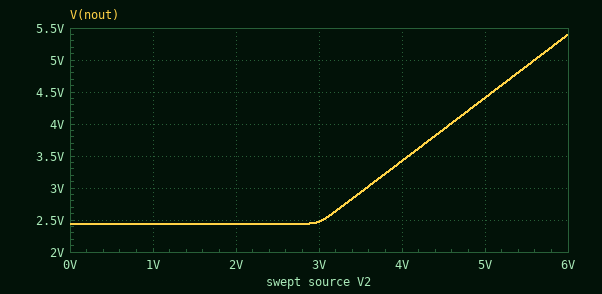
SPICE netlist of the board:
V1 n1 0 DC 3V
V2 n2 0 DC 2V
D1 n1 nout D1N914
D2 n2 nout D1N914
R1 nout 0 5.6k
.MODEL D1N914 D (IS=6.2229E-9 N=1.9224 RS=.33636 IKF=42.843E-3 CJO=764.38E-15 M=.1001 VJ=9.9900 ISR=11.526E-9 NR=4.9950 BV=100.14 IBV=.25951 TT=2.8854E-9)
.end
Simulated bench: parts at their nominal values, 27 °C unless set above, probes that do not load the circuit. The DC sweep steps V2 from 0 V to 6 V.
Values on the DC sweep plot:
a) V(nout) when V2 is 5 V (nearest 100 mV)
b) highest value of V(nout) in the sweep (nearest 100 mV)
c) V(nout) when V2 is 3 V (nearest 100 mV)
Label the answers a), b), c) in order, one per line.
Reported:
a) 4.4 V
b) 5.4 V
c) 2.5 V
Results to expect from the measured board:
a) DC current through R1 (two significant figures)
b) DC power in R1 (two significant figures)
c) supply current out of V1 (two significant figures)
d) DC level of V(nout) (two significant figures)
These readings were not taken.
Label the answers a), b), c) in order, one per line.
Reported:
a) 440 µA
b) 1.1 mW
c) 440 µA
d) 2.4 V
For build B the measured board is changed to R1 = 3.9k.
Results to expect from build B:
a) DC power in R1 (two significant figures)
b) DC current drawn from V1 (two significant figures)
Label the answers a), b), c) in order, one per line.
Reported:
a) 1.5 mW
b) 620 µA
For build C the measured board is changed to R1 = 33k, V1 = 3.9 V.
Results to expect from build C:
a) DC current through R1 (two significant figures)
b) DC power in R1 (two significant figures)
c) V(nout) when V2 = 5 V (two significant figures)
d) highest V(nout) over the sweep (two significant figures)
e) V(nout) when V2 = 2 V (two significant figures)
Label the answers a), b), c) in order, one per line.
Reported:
a) 100 µA
b) 350 µW
c) 4.5 V
d) 5.5 V
e) 3.4 V
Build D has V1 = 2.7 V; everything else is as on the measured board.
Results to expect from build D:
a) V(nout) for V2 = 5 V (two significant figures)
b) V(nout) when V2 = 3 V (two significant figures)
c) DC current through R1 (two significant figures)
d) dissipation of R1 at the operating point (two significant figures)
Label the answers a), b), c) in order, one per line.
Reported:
a) 4.4 V
b) 2.4 V
c) 380 µA
d) 820 µW
